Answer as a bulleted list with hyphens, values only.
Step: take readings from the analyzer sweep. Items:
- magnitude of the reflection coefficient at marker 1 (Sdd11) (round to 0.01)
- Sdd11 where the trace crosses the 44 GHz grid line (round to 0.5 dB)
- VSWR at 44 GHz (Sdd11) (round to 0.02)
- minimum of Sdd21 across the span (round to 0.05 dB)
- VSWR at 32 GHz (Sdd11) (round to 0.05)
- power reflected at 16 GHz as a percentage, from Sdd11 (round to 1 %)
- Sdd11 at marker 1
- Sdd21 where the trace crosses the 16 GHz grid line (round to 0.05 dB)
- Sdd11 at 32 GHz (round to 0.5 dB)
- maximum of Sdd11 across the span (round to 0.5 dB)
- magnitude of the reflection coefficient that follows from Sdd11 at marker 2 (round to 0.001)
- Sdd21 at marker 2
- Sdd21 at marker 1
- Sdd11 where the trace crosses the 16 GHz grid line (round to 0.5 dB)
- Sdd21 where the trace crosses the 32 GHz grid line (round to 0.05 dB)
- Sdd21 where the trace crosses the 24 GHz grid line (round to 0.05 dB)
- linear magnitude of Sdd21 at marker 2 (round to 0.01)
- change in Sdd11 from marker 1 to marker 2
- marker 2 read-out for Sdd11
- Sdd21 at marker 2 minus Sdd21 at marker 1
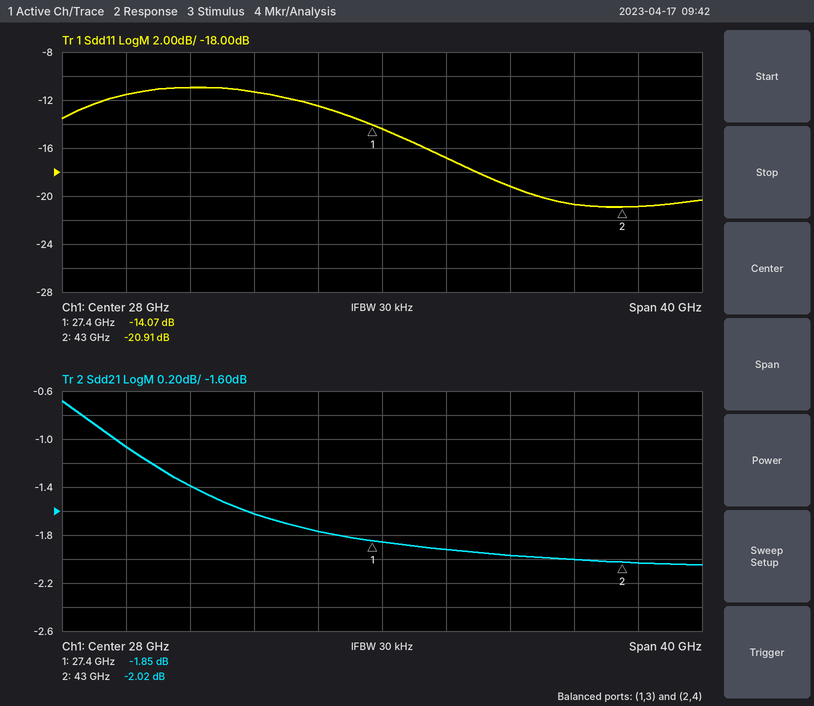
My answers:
- 0.20
- -21.0 dB
- 1.20
- -2.05 dB
- 1.35
- 8 %
- -14.07 dB
- -1.40 dB
- -17.0 dB
- -11.0 dB
- 0.090
- -2.02 dB
- -1.85 dB
- -11.0 dB
- -1.90 dB
- -1.75 dB
- 0.79
- -6.84 dB
- -20.91 dB
- -0.17 dB
